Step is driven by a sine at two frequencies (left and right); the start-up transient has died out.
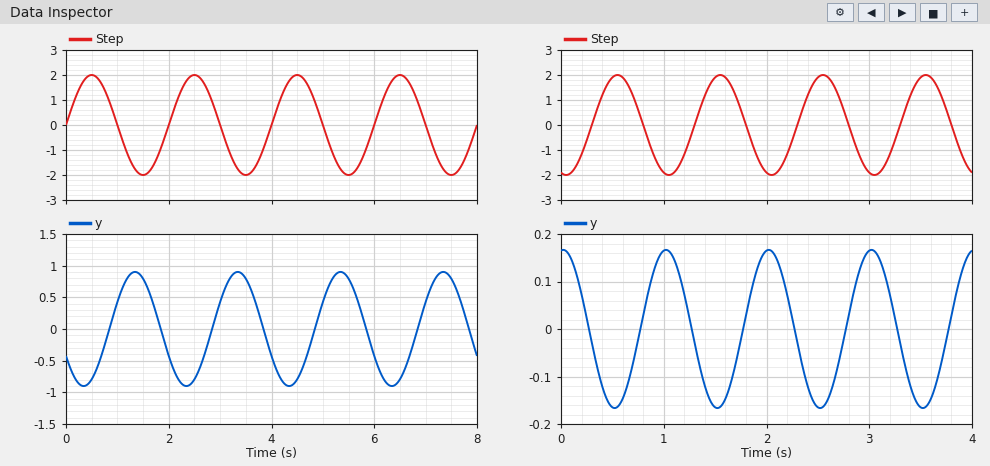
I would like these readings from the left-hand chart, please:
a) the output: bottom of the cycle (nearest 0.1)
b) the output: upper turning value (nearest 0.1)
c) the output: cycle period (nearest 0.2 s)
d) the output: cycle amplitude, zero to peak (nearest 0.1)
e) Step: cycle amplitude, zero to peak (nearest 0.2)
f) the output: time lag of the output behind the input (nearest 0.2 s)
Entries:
-0.9
0.9
2.0 s
0.9
2.0
0.8 s
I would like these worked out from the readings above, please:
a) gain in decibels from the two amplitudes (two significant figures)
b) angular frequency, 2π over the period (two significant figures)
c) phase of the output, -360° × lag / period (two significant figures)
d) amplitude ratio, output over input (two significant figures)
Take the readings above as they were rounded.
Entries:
-6.9 dB
3.1 rad/s
-140°
0.45
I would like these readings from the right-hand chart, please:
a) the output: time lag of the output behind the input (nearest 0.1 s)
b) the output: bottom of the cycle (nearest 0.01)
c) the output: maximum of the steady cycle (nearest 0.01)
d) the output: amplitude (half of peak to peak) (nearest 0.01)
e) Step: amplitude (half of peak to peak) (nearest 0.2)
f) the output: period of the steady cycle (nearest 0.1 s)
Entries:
0.5 s
-0.17
0.17
0.17
2.0
1.0 s
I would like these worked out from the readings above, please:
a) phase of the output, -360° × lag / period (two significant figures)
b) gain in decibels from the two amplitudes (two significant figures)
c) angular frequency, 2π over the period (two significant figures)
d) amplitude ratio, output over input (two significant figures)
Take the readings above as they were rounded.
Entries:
-180°
-21 dB
6.3 rad/s
0.085
